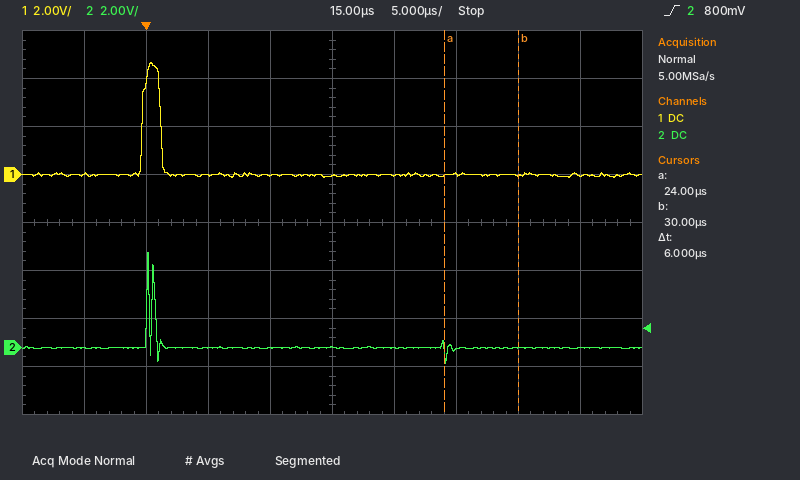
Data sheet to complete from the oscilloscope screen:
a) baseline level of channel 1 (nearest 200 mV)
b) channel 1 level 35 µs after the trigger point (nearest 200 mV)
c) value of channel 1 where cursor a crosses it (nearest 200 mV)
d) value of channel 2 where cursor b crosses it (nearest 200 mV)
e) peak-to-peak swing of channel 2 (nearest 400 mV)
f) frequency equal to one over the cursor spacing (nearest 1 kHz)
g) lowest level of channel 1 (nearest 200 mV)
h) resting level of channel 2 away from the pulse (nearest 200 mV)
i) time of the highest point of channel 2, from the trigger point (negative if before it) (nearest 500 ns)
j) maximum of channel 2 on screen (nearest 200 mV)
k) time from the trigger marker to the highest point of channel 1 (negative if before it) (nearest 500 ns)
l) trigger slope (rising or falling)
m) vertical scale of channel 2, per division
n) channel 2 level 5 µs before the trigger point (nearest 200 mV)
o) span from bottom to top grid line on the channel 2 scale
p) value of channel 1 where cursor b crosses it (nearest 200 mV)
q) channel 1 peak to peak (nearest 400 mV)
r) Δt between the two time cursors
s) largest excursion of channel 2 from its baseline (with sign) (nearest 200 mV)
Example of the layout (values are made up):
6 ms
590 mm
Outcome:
0.0 V
0.0 V
0.0 V
0.0 V
4.8 V
167 kHz
-200 mV
0.0 V
0.0 µs
4.0 V
+500 ns
rising
2 V
0.0 V
16 V
0.0 V
4.8 V
6 µs
+4.0 V
